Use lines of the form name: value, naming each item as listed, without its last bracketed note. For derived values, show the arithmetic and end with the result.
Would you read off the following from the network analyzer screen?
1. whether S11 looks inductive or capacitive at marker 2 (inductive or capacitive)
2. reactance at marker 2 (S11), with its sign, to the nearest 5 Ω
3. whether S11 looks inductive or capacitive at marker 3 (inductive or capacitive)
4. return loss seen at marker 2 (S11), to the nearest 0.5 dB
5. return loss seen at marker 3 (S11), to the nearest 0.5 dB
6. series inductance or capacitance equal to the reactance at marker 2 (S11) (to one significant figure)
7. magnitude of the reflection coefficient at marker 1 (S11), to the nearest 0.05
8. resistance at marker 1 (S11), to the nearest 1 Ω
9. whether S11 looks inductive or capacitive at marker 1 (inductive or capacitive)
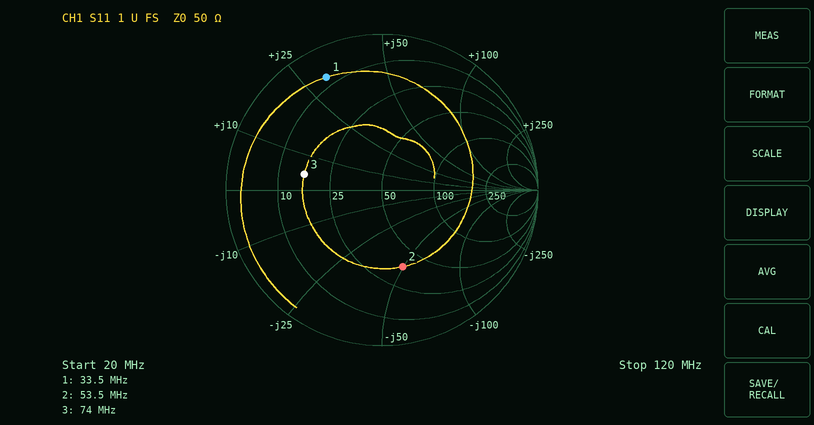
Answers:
whether S11 looks inductive or capacitive at marker 2: capacitive
reactance at marker 2 (S11), with its sign, to the nearest 5 Ω: -50 Ω
whether S11 looks inductive or capacitive at marker 3: inductive
return loss seen at marker 2 (S11), to the nearest 0.5 dB: 6.0 dB
return loss seen at marker 3 (S11), to the nearest 0.5 dB: 6.0 dB
series inductance or capacitance equal to the reactance at marker 2 (S11): C = 1/(2π × 53.5 MHz × 50 Ω) ≈ 60 pF
magnitude of the reflection coefficient at marker 1 (S11), to the nearest 0.05: 0.80
resistance at marker 1 (S11), to the nearest 1 Ω: 7 Ω
whether S11 looks inductive or capacitive at marker 1: inductive
